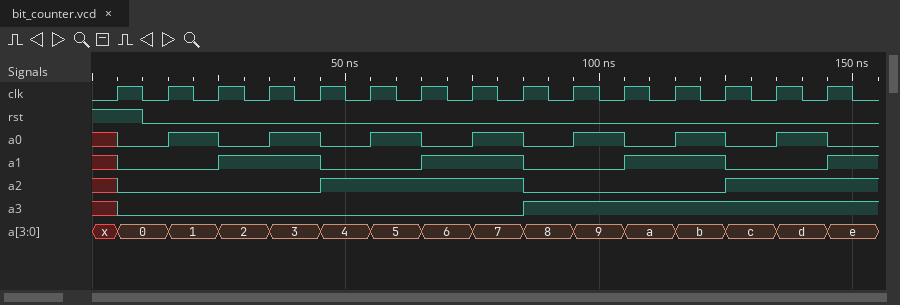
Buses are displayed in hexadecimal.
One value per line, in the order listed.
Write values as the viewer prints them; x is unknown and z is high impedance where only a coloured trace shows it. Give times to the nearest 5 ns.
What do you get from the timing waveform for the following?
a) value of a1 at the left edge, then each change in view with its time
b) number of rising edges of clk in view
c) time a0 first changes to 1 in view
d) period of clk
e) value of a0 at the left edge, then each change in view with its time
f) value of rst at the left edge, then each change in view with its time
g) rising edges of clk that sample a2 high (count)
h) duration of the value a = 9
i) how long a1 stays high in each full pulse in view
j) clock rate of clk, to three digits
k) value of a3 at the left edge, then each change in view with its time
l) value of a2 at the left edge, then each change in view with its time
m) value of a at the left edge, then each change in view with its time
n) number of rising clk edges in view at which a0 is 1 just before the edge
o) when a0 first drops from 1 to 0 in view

x, 0 at 5 ns, 1 at 25 ns, 0 at 45 ns, 1 at 65 ns, 0 at 85 ns, 1 at 105 ns, 0 at 125 ns, 1 at 145 ns
15
15 ns
10 ns
x, 0 at 5 ns, 1 at 15 ns, 0 at 25 ns, 1 at 35 ns, 0 at 45 ns, 1 at 55 ns, 0 at 65 ns, 1 at 75 ns, 0 at 85 ns, 1 at 95 ns, 0 at 105 ns, 1 at 115 ns, 0 at 125 ns, 1 at 135 ns, 0 at 145 ns
1, 0 at 10 ns
6
10 ns
20 ns, 20 ns, 20 ns
100 MHz
x, 0 at 5 ns, 1 at 85 ns
x, 0 at 5 ns, 1 at 45 ns, 0 at 85 ns, 1 at 125 ns
x, 0 at 5 ns, 1 at 15 ns, 2 at 25 ns, 3 at 35 ns, 4 at 45 ns, 5 at 55 ns, 6 at 65 ns, 7 at 75 ns, 8 at 85 ns, 9 at 95 ns, a at 105 ns, b at 115 ns, c at 125 ns, d at 135 ns, e at 145 ns
7
25 ns
